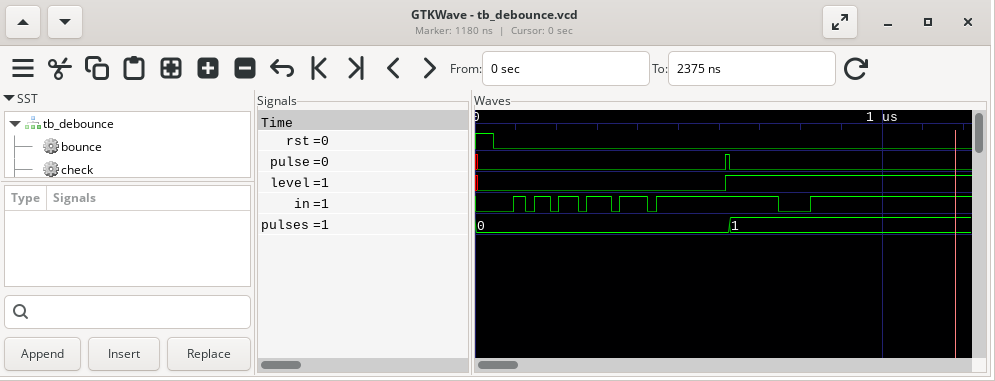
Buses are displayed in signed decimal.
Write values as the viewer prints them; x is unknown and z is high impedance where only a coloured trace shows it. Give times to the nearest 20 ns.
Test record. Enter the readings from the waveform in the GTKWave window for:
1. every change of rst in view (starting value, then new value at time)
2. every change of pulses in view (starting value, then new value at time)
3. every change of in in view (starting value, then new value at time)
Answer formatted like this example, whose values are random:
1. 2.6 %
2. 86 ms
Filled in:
1. 1, 0 at 40 ns
2. 0, 1 at 620 ns
3. 0, 1 at 100 ns, 0 at 120 ns, 1 at 140 ns, 0 at 180 ns, 1 at 200 ns, 0 at 260 ns, 1 at 280 ns, 0 at 340 ns, 1 at 360 ns, 0 at 420 ns, 1 at 440 ns, 0 at 740 ns, 1 at 820 ns
